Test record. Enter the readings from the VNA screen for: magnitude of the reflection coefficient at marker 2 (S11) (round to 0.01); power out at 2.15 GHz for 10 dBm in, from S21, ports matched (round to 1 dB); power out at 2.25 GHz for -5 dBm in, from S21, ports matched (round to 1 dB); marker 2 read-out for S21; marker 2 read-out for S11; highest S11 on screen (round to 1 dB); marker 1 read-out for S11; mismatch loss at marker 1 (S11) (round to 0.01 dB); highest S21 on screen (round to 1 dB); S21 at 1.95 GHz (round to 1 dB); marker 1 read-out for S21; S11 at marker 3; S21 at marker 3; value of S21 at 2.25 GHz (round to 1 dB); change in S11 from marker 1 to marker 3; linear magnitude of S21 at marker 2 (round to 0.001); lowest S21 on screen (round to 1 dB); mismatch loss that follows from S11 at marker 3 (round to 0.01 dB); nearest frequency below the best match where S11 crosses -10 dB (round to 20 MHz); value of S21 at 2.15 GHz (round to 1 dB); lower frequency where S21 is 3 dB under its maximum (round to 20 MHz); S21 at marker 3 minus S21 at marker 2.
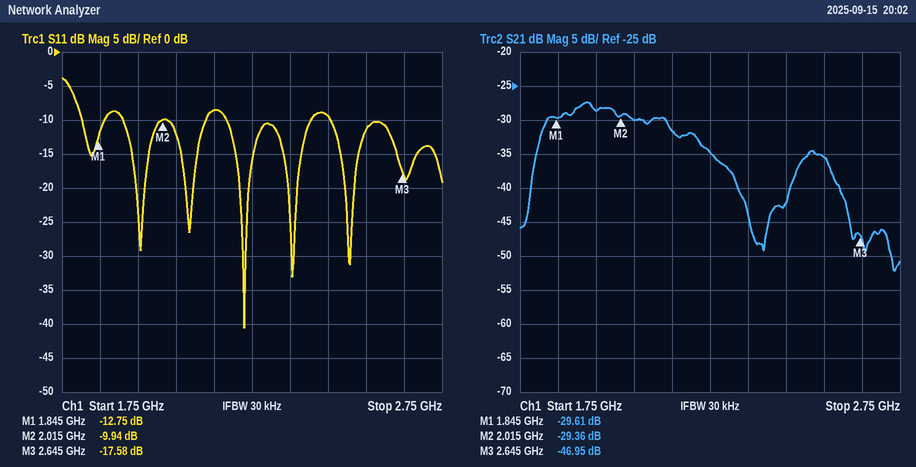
0.32
-22 dBm
-40 dBm
-29.36 dB
-9.94 dB
-4 dB
-12.75 dB
0.24 dB
-27 dB
-29 dB
-29.61 dB
-17.58 dB
-46.95 dB
-35 dB
-4.83 dB
0.034
-52 dB
0.08 dB
2.18 GHz
-32 dB
1.82 GHz
-17.59 dB
